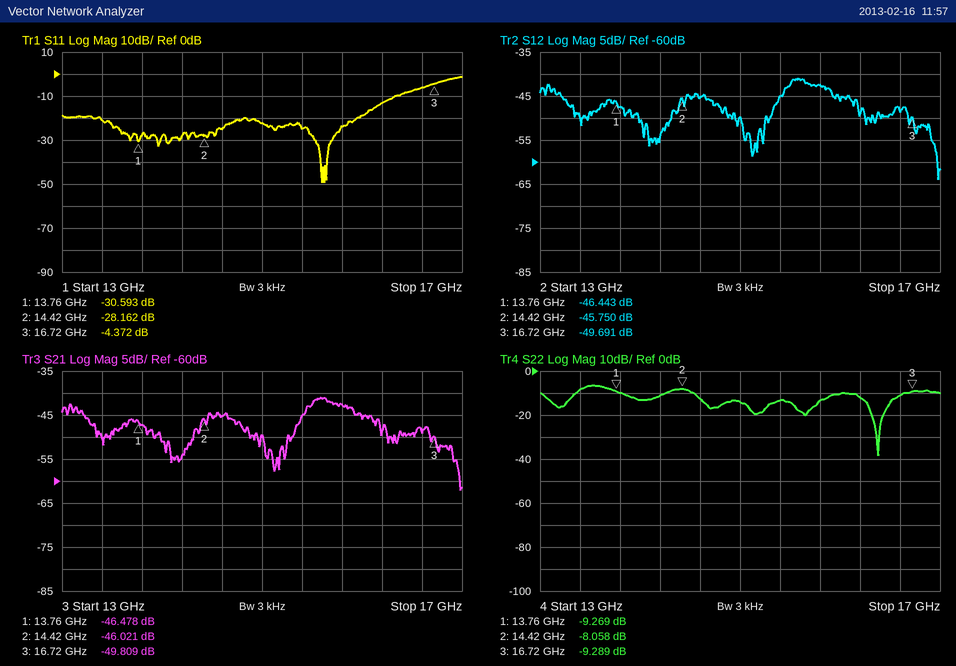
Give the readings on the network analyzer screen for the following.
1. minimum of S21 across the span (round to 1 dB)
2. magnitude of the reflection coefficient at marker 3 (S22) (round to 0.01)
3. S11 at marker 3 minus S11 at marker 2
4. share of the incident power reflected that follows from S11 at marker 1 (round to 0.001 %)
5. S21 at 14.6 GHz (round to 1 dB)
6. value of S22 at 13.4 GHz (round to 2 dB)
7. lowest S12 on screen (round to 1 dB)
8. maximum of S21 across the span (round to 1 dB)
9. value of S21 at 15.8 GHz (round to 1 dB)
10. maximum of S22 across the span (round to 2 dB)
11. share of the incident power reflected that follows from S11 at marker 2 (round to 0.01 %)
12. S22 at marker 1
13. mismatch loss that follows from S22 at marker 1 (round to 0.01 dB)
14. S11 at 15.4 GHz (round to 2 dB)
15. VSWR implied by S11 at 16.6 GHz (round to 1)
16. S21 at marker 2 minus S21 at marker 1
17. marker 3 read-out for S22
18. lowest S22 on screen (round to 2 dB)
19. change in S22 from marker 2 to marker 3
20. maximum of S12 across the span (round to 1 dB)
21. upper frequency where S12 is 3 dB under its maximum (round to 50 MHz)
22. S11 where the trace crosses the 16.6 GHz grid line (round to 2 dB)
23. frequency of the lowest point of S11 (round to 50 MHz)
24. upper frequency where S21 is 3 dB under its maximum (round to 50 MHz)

-62 dB
0.34
23.790 dB
0.087 %
-45 dB
-8 dB
-64 dB
-41 dB
-43 dB
-6 dB
0.15 %
-9.269 dB
0.55 dB
-24 dB
3
0.457 dB
-9.289 dB
-38 dB
-1.231 dB
-41 dB
15.90 GHz
-6 dB
15.60 GHz
15.90 GHz
